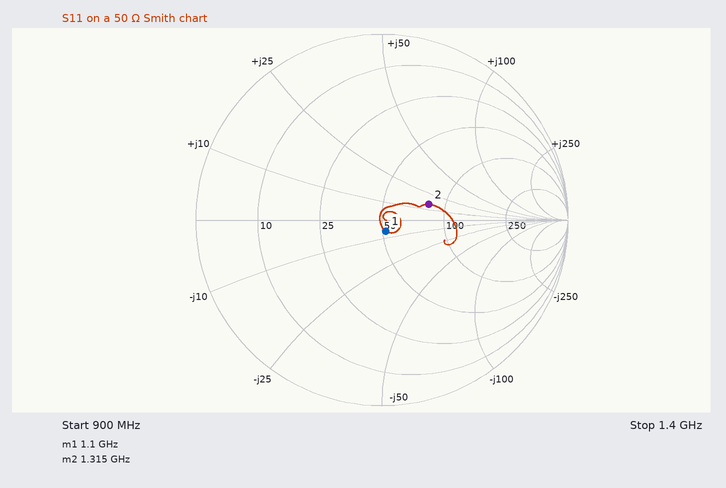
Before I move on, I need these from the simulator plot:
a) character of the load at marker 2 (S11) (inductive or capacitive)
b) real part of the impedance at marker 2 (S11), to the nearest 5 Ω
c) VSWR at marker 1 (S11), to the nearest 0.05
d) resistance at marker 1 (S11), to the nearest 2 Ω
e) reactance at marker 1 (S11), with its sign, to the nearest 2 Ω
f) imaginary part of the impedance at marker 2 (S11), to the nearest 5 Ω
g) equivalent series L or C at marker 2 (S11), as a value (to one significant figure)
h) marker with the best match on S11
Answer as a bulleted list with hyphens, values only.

- inductive
- 80 Ω
- 1.15
- 52 Ω
- -6 Ω
- +15 Ω
- 2 nH
- marker 1
